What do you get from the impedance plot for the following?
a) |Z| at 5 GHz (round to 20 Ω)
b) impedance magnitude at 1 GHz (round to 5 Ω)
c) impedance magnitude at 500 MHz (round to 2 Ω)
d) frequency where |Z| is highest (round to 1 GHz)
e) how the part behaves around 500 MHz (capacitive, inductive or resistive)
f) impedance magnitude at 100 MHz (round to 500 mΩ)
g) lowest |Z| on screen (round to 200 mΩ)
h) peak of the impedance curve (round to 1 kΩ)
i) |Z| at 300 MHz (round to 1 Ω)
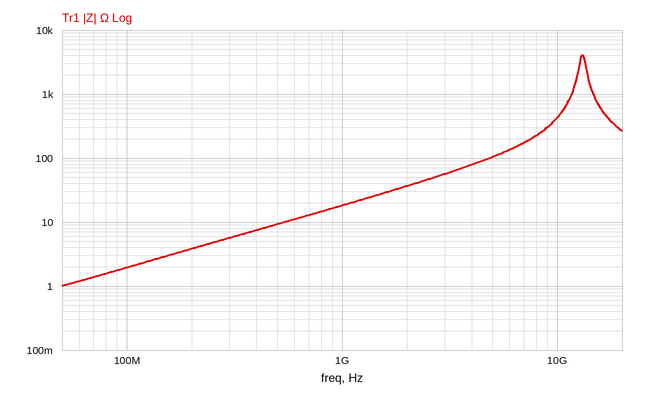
100 Ω
20 Ω
10 Ω
13 GHz
inductive
2.0 Ω
1.0 Ω
4 kΩ
6 Ω
